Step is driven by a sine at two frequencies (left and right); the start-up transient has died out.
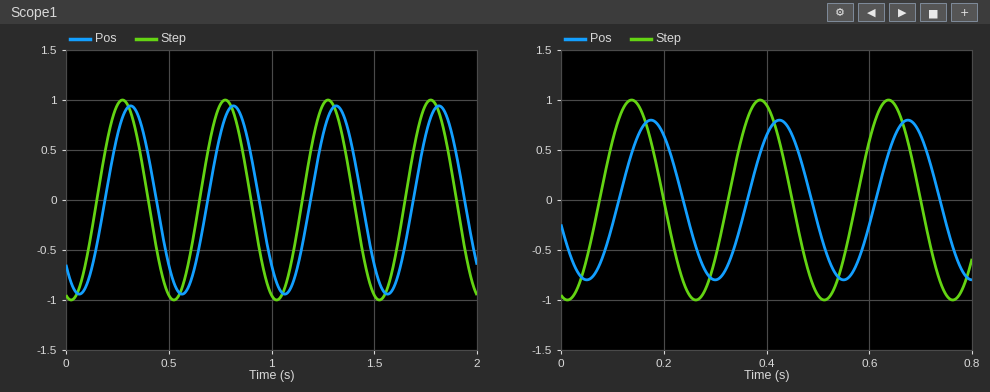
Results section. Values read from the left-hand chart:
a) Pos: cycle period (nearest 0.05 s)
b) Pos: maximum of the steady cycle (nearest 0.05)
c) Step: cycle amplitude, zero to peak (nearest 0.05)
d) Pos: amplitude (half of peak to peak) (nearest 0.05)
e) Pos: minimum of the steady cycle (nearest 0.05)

0.50 s
0.95
1.00
0.95
-0.95
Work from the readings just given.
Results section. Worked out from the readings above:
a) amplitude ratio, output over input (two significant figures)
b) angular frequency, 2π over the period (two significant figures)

0.95
13 rad/s
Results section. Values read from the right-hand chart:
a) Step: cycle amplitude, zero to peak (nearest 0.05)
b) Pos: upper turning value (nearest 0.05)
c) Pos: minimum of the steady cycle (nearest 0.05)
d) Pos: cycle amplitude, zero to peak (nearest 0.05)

1.00
0.80
-0.80
0.80
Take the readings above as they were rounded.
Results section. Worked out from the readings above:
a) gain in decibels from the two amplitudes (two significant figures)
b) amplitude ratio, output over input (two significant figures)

-1.9 dB
0.80
